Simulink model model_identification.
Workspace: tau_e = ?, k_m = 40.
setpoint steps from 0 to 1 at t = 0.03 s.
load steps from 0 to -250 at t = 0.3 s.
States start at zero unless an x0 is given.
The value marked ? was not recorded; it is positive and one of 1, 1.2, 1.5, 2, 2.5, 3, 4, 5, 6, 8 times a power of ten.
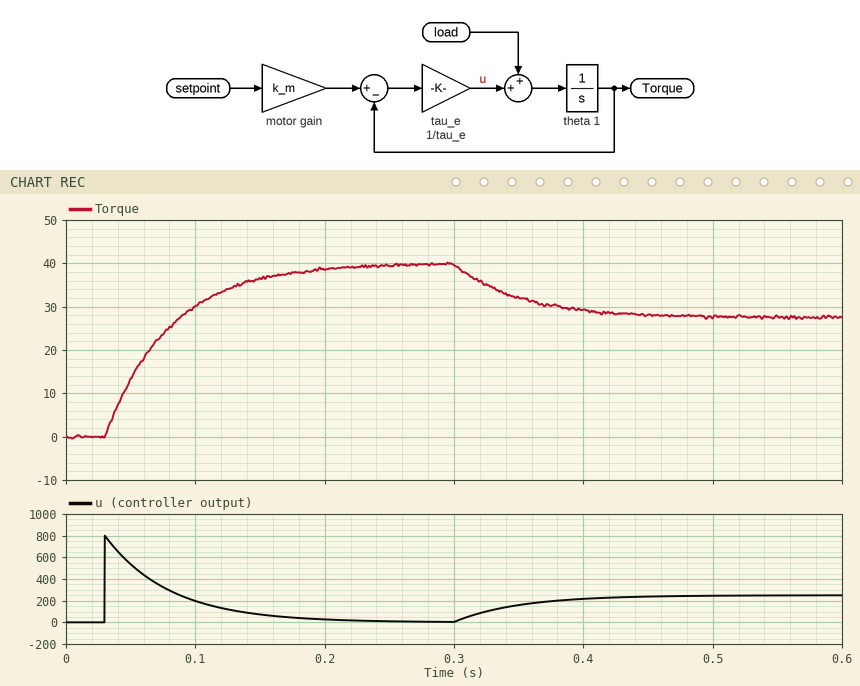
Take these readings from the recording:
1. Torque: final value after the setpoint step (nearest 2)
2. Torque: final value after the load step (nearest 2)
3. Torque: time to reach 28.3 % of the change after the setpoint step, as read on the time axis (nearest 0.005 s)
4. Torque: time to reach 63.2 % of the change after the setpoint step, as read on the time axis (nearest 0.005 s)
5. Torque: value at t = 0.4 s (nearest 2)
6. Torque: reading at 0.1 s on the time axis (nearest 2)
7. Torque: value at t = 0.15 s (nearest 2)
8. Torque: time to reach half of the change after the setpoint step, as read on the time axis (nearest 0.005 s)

40
28
0.045 s
0.080 s
30
30
36
0.065 s
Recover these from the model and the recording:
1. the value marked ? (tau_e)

0.05
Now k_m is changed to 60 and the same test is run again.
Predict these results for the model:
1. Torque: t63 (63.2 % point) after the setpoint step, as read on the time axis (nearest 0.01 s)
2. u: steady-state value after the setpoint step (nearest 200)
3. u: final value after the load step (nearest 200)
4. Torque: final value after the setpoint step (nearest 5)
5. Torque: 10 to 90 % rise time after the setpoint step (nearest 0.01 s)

0.08 s
0
200
60
0.11 s
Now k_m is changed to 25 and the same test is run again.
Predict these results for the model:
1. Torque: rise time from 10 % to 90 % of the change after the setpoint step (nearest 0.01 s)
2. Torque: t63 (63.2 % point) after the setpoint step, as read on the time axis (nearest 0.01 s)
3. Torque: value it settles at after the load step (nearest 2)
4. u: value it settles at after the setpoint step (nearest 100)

0.11 s
0.08 s
12
0
